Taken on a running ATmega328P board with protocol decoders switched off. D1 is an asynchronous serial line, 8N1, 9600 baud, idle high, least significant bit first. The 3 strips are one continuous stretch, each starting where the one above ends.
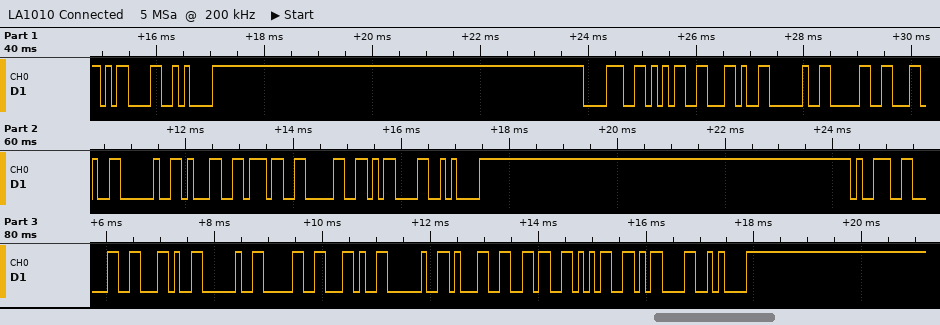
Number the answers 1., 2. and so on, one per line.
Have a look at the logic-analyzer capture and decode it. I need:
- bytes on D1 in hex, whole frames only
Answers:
1. 0D 0A 38 35 2C 20 30 2C 20 31 37 30 0D 0A 39 30 2C 20 30 2C 20 31 36 35 0D 0A
